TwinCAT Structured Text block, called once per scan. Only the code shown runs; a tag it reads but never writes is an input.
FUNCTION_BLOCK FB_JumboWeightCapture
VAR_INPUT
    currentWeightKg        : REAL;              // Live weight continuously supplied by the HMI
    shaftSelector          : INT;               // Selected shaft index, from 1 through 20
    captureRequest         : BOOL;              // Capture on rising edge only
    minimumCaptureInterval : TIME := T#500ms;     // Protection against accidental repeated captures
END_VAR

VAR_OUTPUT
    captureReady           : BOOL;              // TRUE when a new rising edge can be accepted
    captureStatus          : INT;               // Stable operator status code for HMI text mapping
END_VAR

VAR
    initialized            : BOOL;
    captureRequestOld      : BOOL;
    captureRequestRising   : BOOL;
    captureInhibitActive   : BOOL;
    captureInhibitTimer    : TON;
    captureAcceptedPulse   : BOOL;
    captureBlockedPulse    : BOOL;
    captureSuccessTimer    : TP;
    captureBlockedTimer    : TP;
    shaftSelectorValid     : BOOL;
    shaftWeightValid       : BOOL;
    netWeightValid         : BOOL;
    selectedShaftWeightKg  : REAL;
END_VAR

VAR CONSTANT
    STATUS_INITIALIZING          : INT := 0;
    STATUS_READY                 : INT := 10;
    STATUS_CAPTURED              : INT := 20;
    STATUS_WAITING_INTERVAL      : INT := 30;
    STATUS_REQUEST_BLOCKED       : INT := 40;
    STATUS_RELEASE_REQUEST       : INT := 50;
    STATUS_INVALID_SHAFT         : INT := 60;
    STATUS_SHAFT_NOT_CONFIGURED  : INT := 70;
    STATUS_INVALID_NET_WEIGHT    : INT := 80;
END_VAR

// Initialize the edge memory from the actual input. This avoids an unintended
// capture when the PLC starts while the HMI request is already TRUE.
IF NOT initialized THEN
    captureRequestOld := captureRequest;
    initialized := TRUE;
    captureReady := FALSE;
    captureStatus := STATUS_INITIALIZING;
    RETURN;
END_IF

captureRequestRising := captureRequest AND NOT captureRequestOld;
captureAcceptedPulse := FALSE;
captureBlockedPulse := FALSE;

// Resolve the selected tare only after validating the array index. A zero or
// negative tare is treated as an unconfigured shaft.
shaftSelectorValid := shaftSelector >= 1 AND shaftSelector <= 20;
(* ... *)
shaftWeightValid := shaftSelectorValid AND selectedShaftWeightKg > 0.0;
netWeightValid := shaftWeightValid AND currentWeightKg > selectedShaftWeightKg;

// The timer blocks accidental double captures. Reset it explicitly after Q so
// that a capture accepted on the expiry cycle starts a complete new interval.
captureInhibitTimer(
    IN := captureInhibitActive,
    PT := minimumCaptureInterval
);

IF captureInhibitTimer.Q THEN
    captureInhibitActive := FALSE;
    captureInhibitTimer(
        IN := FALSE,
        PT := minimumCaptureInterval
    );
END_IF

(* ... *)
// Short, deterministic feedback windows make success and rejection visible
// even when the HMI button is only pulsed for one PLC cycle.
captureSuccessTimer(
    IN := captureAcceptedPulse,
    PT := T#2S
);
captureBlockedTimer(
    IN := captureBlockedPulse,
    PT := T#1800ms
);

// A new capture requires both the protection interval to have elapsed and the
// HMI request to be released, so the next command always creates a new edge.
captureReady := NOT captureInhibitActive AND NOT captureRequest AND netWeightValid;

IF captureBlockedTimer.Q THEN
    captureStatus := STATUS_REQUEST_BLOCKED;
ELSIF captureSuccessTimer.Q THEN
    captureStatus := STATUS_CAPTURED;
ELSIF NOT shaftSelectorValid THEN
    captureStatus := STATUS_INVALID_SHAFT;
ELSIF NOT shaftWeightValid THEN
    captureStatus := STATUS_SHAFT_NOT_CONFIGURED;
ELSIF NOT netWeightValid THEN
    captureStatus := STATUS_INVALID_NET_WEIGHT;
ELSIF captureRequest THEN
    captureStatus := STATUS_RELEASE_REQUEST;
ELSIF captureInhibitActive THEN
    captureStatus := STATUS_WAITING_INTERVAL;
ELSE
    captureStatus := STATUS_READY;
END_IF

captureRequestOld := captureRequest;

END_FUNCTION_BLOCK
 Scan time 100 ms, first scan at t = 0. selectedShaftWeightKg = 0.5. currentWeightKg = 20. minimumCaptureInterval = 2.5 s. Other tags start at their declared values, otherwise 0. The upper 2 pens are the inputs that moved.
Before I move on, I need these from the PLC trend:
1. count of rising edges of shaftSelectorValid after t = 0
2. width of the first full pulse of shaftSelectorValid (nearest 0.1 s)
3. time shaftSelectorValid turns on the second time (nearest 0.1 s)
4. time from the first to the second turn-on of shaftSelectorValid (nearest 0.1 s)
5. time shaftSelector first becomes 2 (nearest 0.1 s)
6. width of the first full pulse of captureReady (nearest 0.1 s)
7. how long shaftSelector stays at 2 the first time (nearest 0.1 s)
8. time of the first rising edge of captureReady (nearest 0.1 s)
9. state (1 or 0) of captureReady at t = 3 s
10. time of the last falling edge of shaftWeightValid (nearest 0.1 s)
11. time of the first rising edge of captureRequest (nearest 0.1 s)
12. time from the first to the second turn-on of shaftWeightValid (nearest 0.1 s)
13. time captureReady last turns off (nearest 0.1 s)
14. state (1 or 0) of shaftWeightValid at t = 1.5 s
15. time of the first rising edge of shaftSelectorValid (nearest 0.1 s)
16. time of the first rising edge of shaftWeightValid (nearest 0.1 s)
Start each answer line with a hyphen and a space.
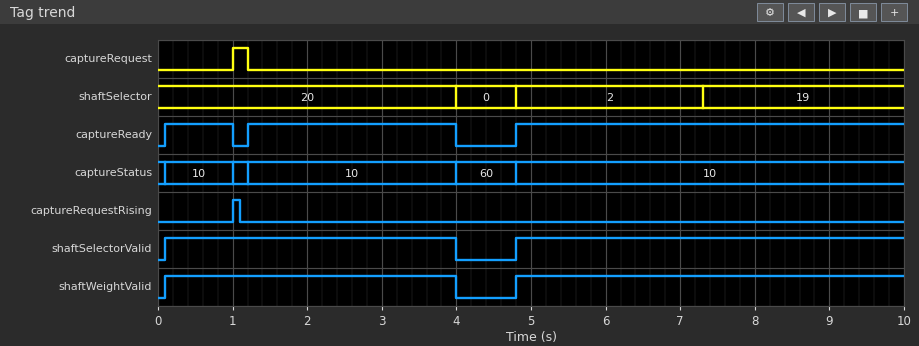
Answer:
- 2
- 3.9 s
- 4.8 s
- 4.7 s
- 4.8 s
- 0.9 s
- 2.5 s
- 0.1 s
- 1
- 4.0 s
- 1.0 s
- 4.7 s
- 4.0 s
- 1
- 0.1 s
- 0.1 s
